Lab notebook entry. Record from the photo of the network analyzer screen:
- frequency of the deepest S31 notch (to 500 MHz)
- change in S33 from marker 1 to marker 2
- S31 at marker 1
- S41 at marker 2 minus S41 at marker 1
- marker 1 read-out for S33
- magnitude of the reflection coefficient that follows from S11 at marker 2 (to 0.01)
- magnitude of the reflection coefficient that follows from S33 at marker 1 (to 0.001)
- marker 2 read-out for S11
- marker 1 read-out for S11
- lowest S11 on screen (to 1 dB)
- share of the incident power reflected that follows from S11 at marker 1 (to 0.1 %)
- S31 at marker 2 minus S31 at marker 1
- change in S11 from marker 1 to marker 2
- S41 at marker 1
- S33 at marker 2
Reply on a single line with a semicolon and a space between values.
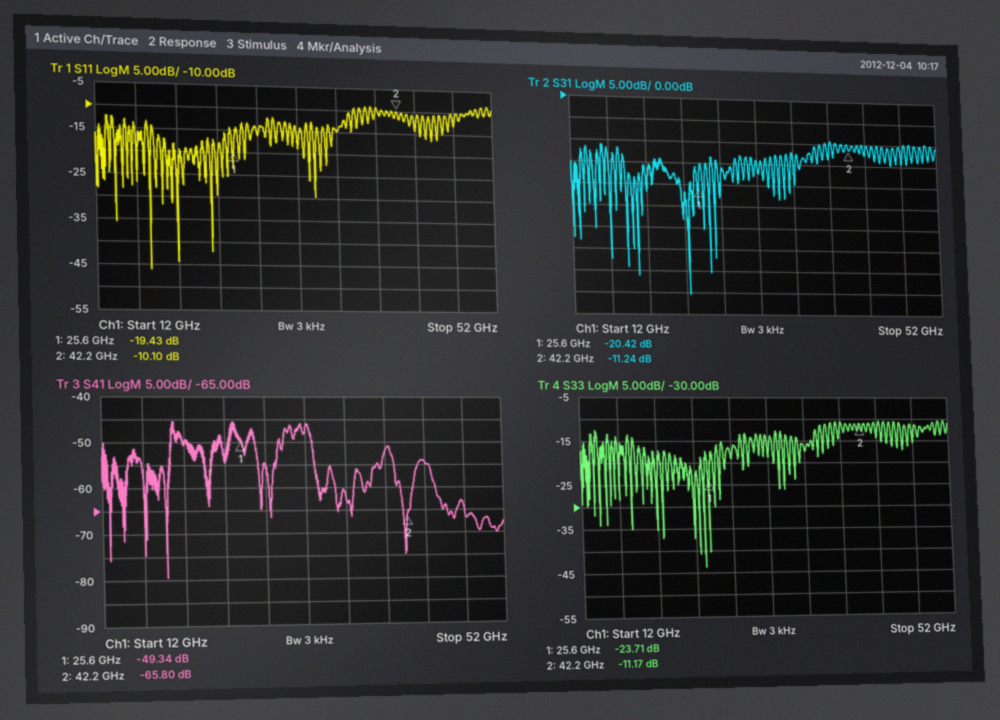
24.5 GHz; 12.54 dB; -20.42 dB; -16.46 dB; -23.71 dB; 0.31; 0.065; -10.10 dB; -19.43 dB; -46 dB; 1.1 %; 9.18 dB; 9.33 dB; -49.34 dB; -11.17 dB
